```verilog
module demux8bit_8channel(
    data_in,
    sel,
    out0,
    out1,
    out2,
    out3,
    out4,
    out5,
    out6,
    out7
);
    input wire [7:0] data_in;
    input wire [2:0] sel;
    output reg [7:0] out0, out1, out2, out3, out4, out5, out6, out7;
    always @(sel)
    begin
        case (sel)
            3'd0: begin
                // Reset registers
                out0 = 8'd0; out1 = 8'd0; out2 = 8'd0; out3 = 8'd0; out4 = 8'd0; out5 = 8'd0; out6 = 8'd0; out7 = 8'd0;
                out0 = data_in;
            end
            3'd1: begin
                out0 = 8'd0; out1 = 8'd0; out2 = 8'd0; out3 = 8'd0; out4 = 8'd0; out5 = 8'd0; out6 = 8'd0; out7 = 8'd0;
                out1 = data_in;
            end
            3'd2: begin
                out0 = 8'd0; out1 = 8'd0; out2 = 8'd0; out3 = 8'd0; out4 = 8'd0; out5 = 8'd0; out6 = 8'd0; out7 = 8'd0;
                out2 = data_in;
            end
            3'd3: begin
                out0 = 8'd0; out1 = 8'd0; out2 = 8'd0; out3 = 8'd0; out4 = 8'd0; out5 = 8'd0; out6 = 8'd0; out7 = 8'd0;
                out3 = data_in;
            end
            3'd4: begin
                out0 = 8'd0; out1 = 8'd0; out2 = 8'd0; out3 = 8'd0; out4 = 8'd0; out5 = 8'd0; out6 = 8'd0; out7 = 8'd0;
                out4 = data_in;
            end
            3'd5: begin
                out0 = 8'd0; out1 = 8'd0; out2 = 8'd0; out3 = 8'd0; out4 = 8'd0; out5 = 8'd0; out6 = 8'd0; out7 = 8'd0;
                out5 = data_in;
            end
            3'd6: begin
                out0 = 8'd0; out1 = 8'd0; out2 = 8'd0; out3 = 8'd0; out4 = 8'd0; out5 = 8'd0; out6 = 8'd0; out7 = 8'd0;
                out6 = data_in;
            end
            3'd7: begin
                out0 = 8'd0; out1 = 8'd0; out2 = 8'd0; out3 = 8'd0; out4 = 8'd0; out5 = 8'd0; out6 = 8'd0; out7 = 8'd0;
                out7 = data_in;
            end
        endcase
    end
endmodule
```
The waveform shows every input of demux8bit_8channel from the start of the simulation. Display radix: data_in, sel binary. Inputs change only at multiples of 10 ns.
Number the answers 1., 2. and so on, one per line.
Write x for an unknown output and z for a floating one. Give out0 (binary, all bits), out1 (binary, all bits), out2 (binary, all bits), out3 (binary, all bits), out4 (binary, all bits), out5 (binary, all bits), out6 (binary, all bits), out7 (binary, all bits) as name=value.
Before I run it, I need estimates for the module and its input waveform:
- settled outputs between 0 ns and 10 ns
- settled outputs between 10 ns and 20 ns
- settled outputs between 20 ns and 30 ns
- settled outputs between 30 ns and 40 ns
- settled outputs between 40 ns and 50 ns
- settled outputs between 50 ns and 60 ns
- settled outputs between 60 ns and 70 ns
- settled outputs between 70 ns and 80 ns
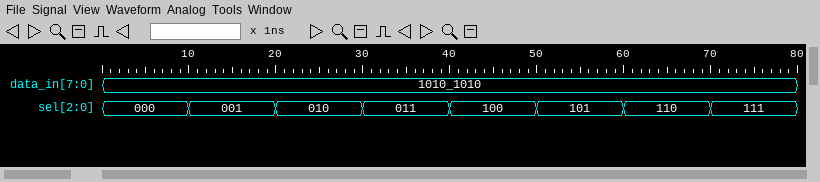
1. out0=10101010, out1=00000000, out2=00000000, out3=00000000, out4=00000000, out5=00000000, out6=00000000, out7=00000000
2. out0=00000000, out1=10101010, out2=00000000, out3=00000000, out4=00000000, out5=00000000, out6=00000000, out7=00000000
3. out0=00000000, out1=00000000, out2=10101010, out3=00000000, out4=00000000, out5=00000000, out6=00000000, out7=00000000
4. out0=00000000, out1=00000000, out2=00000000, out3=10101010, out4=00000000, out5=00000000, out6=00000000, out7=00000000
5. out0=00000000, out1=00000000, out2=00000000, out3=00000000, out4=10101010, out5=00000000, out6=00000000, out7=00000000
6. out0=00000000, out1=00000000, out2=00000000, out3=00000000, out4=00000000, out5=10101010, out6=00000000, out7=00000000
7. out0=00000000, out1=00000000, out2=00000000, out3=00000000, out4=00000000, out5=00000000, out6=10101010, out7=00000000
8. out0=00000000, out1=00000000, out2=00000000, out3=00000000, out4=00000000, out5=00000000, out6=00000000, out7=10101010
